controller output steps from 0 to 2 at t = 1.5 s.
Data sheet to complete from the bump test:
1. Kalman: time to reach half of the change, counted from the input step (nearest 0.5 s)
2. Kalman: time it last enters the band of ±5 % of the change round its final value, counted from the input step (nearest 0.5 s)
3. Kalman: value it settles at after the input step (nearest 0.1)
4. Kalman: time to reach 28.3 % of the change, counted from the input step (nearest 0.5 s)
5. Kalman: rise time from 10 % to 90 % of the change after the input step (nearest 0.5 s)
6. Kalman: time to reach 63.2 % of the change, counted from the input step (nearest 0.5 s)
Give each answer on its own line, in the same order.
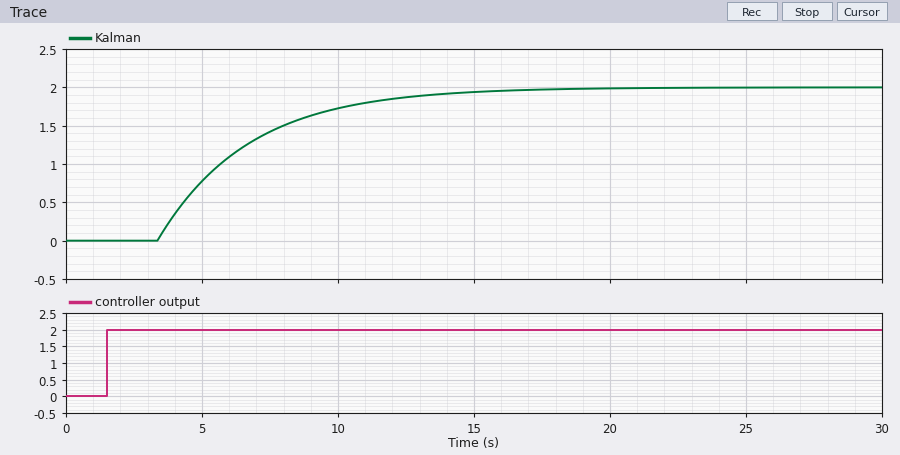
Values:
4.0 s
12.0 s
2.0
3.0 s
7.5 s
5.0 s
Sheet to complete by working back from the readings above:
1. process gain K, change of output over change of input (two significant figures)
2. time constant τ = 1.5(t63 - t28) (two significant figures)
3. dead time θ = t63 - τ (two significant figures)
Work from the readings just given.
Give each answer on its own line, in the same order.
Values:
1.0
3.0 s
2.0 s
